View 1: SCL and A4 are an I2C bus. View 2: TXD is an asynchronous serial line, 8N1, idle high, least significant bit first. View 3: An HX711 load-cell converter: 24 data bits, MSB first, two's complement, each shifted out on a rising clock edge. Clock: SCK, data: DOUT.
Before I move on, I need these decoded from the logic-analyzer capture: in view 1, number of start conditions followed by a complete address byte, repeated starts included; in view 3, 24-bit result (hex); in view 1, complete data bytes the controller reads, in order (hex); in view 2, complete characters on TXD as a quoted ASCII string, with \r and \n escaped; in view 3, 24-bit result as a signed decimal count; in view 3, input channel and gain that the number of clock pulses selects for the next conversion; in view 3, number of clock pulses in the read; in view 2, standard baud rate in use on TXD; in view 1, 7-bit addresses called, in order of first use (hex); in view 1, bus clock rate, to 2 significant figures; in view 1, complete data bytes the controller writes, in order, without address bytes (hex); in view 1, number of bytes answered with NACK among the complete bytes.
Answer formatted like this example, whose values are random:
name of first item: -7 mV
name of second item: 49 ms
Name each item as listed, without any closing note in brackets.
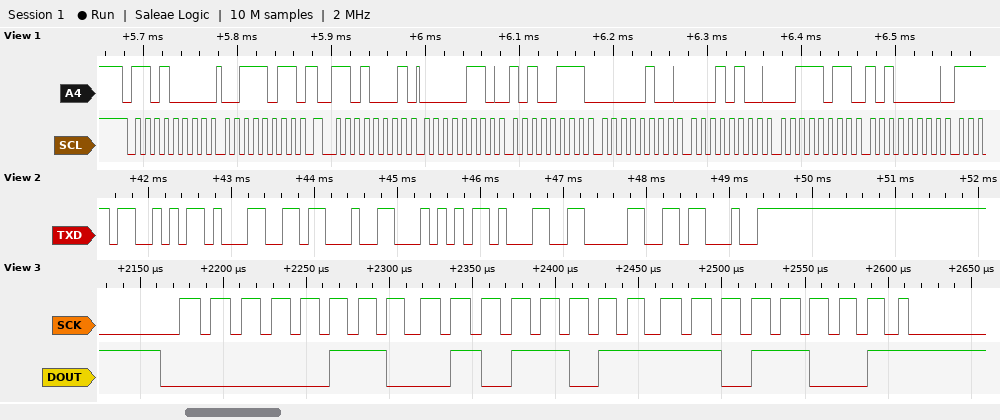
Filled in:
in view 1, number of start conditions followed by a complete address byte, repeated starts included: 2
in view 3, 24-bit result: 0x065BD9
in view 1, complete data bytes the controller reads, in order: 06 A7 04 14 3B A0
in view 2, complete characters on TXD as a quoted ASCII string, with \r and \n escaped: "S1#T10#"
in view 3, 24-bit result as a signed decimal count: 416729
in view 3, input channel and gain that the number of clock pulses selects for the next conversion: channel A, gain 128
in view 3, number of clock pulses in the read: 25
in view 2, standard baud rate in use on TXD: 9600 baud
in view 1, 7-bit addresses called, in order of first use: 0x68
in view 1, bus clock rate, to 2 significant figures: 100 kHz
in view 1, complete data bytes the controller writes, in order, without address bytes: 3B
in view 1, number of bytes answered with NACK among the complete bytes: 0
